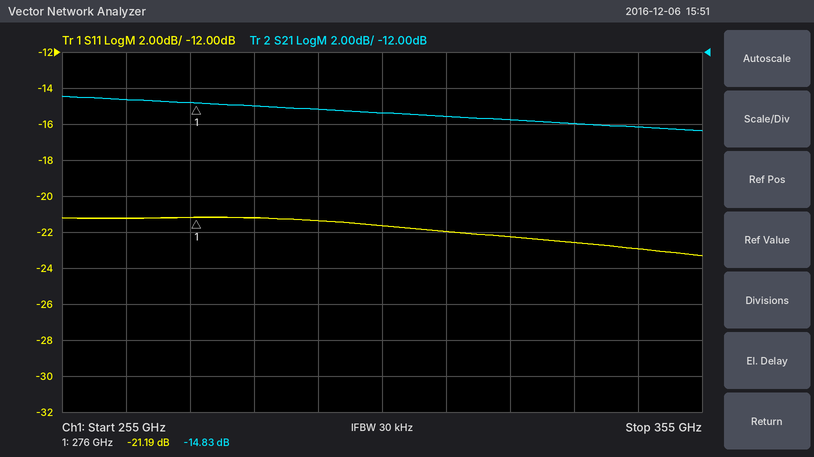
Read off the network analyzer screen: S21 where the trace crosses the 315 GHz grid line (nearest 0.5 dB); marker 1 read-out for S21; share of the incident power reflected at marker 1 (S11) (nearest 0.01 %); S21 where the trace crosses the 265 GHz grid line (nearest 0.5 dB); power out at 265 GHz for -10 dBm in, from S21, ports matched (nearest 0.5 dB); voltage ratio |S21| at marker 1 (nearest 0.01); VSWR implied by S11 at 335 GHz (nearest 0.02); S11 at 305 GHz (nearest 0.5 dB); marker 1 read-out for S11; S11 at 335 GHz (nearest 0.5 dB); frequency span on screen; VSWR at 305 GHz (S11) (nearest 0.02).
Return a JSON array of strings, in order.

["-15.5 dB", "-14.83 dB", "0.76 %", "-14.5 dB", "-24.5 dBm", "0.18", "1.16", "-21.5 dB", "-21.19 dB", "-22.5 dB", "100 GHz", "1.18"]
